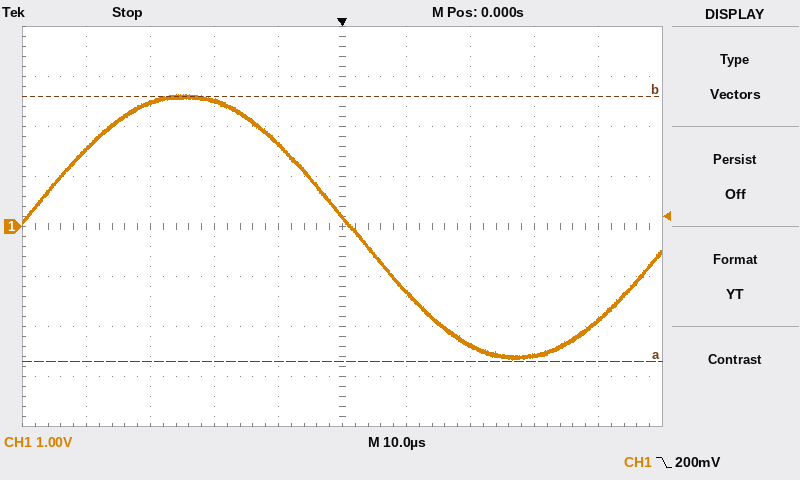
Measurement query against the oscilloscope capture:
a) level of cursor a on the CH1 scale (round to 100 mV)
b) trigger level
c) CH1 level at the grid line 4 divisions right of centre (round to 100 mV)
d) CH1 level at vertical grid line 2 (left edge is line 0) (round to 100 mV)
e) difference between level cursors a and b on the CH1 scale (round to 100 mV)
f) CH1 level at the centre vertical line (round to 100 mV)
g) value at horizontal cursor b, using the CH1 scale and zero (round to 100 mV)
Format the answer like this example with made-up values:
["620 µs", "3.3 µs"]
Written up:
["-2.7 V", "200 mV", "-1.9 V", "2.5 V", "5.3 V", "200 mV", "2.6 V"]
